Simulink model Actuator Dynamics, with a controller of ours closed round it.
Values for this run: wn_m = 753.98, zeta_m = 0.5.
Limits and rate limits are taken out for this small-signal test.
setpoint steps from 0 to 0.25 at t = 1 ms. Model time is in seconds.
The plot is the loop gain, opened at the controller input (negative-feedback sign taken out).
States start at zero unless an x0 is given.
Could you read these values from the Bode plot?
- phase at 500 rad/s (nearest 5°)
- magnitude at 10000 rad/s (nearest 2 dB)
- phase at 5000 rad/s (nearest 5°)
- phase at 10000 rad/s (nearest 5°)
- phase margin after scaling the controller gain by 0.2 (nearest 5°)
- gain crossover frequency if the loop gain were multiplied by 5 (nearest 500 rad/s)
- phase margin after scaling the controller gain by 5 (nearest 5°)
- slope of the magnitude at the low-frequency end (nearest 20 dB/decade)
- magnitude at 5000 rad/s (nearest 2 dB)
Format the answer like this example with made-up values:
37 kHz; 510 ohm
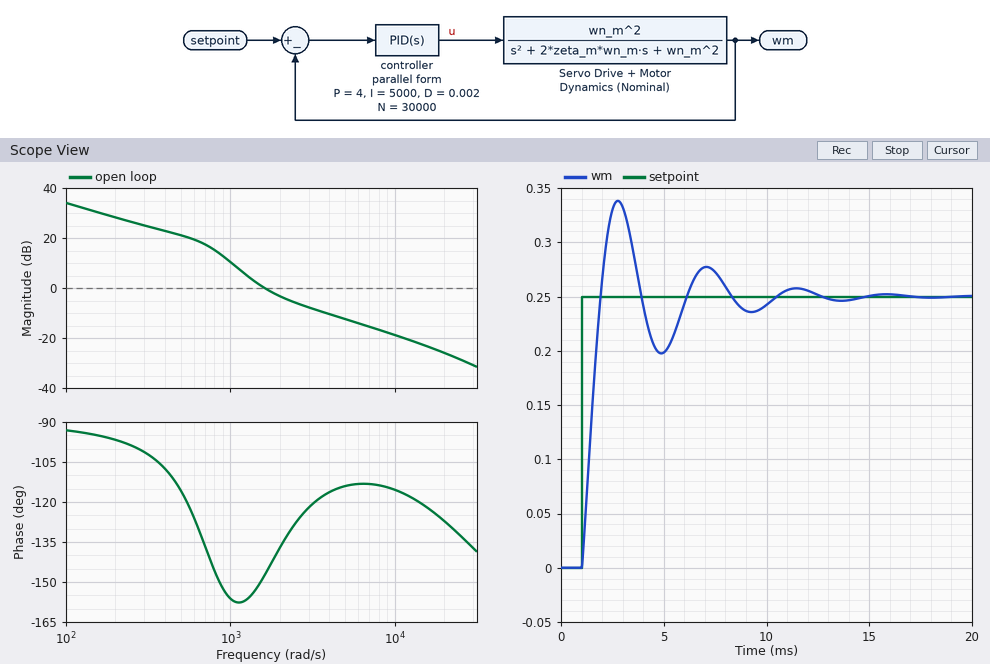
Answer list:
-115°; -18 dB; -115°; -115°; 30°; 6000 rad/s; 65°; -20 dB/decade; -12 dB
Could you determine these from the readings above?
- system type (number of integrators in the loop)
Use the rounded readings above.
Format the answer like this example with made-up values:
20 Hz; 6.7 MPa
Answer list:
1
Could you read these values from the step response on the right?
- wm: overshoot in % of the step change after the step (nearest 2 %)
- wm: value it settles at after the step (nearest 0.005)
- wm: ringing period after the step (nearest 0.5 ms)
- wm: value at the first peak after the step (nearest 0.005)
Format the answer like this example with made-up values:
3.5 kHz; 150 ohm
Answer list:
36 %; 0.250; 4.5 ms; 0.340
